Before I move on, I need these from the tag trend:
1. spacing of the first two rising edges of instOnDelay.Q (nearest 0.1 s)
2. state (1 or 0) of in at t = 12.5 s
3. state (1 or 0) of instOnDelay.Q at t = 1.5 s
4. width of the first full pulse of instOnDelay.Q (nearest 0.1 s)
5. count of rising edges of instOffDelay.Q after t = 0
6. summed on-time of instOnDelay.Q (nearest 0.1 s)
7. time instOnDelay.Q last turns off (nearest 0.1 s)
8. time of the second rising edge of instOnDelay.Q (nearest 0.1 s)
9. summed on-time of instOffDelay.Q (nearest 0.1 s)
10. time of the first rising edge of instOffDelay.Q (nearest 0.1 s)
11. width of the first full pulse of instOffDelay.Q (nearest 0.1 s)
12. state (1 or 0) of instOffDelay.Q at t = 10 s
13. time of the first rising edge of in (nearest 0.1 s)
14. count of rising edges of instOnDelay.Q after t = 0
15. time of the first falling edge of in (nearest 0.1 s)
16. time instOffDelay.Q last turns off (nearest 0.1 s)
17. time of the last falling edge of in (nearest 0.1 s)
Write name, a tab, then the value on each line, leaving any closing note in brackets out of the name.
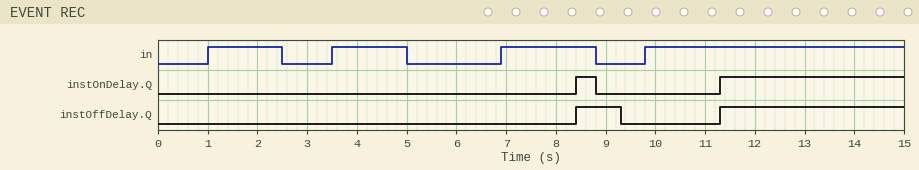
spacing of the first two rising edges of instOnDelay.Q	2.9 s
state (1 or 0) of in at t = 12.5 s	1
state (1 or 0) of instOnDelay.Q at t = 1.5 s	0
width of the first full pulse of instOnDelay.Q	0.4 s
count of rising edges of instOffDelay.Q after t = 0	2
summed on-time of instOnDelay.Q	4.1 s
time instOnDelay.Q last turns off	8.8 s
time of the second rising edge of instOnDelay.Q	11.3 s
summed on-time of instOffDelay.Q	4.6 s
time of the first rising edge of instOffDelay.Q	8.4 s
width of the first full pulse of instOffDelay.Q	0.9 s
state (1 or 0) of instOffDelay.Q at t = 10 s	0
time of the first rising edge of in	1.0 s
count of rising edges of instOnDelay.Q after t = 0	2
time of the first falling edge of in	2.5 s
time instOffDelay.Q last turns off	9.3 s
time of the last falling edge of in	8.8 s
